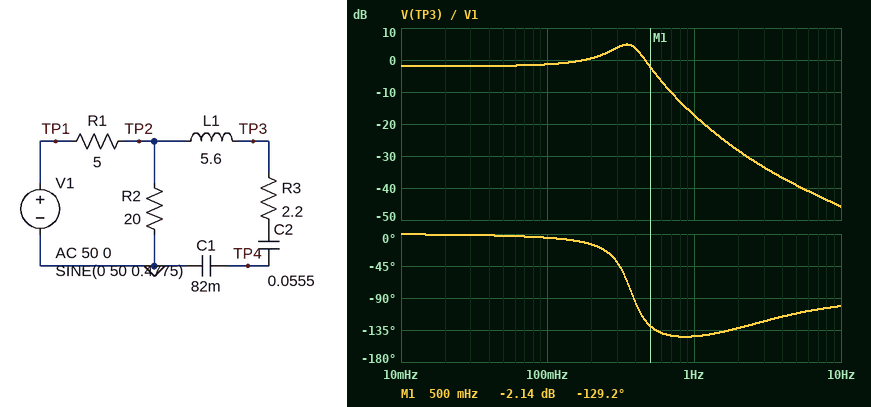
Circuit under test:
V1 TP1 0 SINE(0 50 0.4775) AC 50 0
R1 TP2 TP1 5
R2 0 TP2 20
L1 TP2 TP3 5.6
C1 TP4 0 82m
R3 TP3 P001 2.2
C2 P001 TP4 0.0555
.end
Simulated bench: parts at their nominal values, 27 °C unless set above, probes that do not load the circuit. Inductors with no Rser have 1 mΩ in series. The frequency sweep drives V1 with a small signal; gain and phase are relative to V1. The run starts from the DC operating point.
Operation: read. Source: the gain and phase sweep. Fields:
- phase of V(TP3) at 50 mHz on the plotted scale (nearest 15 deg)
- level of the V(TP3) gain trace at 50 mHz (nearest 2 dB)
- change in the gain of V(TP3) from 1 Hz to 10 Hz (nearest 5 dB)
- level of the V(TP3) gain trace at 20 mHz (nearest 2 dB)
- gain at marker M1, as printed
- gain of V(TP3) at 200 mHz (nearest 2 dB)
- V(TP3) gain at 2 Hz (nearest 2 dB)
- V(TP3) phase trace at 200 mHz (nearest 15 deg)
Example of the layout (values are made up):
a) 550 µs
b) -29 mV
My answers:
a) 0 deg
b) -2 dB
c) -30 dB
d) -2 dB
e) -2.14 dB
f) 0 dB
g) -28 dB
h) -15 deg
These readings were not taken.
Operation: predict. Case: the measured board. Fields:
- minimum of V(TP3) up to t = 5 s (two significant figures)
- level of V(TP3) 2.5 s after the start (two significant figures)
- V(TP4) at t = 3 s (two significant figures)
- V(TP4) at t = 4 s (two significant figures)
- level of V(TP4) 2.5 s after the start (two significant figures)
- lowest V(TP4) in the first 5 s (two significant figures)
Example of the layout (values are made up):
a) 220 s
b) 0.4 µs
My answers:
a) -53 V
b) -36 V
c) 9.4 V
d) -3.5 V
e) -17 V
f) -21 V
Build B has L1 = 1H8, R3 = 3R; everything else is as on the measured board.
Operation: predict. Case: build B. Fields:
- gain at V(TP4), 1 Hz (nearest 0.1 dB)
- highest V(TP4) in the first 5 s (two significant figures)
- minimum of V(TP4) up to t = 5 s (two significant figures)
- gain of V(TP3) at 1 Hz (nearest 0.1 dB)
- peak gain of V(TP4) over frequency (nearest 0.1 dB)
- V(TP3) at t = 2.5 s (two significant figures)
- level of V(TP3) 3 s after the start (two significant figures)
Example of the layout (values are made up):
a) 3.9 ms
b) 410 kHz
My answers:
a) -15.8 dB
b) 19 V
c) -19 V
d) -6.5 dB
e) -8.3 dB
f) 25 V
g) 45 V
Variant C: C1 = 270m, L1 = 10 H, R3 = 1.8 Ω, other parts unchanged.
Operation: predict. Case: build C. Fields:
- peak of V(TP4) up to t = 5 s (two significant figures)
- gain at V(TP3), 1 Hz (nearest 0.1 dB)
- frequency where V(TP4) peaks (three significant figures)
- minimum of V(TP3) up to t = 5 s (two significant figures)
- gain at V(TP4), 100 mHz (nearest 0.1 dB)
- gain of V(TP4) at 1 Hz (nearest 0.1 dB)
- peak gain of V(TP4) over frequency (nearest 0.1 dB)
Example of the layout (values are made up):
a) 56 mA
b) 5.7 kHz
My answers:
a) 4.5 V
b) -25.6 dB
c) 225 mHz
d) -21 V
e) -15.7 dB
f) -42.0 dB
g) -9.0 dB
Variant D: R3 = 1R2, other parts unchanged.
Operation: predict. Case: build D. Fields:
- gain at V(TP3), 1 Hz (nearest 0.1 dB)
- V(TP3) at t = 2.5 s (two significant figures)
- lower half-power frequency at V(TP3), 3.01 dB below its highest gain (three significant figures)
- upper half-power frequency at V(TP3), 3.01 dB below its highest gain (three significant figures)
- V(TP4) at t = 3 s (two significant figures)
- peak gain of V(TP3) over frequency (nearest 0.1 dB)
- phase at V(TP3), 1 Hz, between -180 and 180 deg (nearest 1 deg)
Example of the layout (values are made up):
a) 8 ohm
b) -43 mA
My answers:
a) -17.8 dB
b) -44 V
c) 269 mHz
d) 424 mHz
e) 9.8 V
f) 6.2 dB
g) -156 deg
